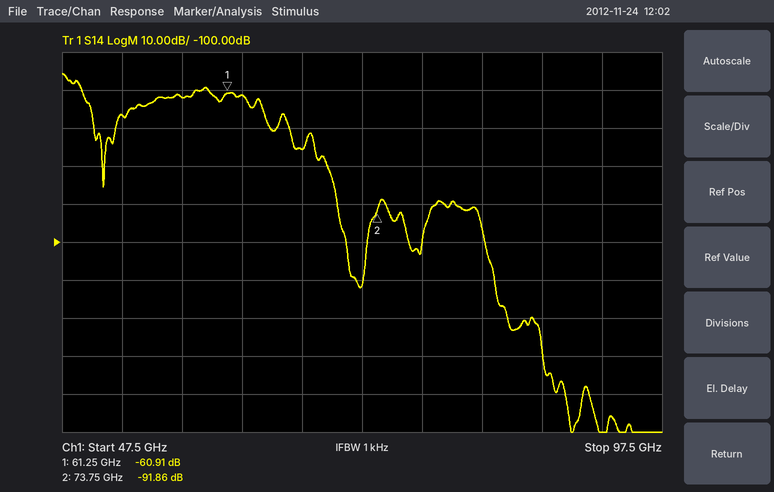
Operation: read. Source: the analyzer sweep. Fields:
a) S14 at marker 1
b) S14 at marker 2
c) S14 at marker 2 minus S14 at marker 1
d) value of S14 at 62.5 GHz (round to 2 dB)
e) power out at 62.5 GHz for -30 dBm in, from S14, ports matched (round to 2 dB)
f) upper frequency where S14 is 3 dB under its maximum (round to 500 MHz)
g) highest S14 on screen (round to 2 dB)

-60.91 dB
-91.86 dB
-30.95 dB
-62 dB
-92 dBm
49.0 GHz
-56 dB
